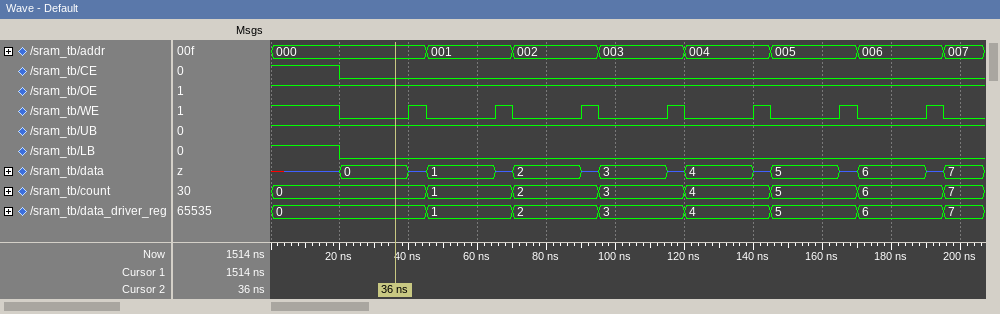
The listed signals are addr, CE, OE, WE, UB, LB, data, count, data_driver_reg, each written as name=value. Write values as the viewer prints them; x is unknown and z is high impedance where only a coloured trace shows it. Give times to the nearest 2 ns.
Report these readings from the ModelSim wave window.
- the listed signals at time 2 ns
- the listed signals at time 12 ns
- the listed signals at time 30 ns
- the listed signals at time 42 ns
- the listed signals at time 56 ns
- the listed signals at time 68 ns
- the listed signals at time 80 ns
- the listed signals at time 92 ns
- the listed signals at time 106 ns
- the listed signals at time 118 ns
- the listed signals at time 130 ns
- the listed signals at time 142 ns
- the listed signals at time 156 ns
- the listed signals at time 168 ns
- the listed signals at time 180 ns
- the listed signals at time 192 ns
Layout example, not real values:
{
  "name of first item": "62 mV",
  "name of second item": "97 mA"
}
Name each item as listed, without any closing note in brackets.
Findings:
{
  "the listed signals at time 2 ns": "addr=000, CE=1, OE=1, WE=1, UB=1, LB=1, data=x, count=0, data_driver_reg=0",
  "the listed signals at time 12 ns": "addr=000, CE=1, OE=1, WE=1, UB=1, LB=1, data=z, count=0, data_driver_reg=0",
  "the listed signals at time 30 ns": "addr=000, CE=0, OE=1, WE=0, UB=1, LB=0, data=0, count=0, data_driver_reg=0",
  "the listed signals at time 42 ns": "addr=000, CE=0, OE=1, WE=1, UB=1, LB=0, data=z, count=0, data_driver_reg=0",
  "the listed signals at time 56 ns": "addr=001, CE=0, OE=1, WE=0, UB=1, LB=0, data=1, count=1, data_driver_reg=1",
  "the listed signals at time 68 ns": "addr=001, CE=0, OE=1, WE=1, UB=1, LB=0, data=z, count=1, data_driver_reg=1",
  "the listed signals at time 80 ns": "addr=002, CE=0, OE=1, WE=0, UB=1, LB=0, data=2, count=2, data_driver_reg=2",
  "the listed signals at time 92 ns": "addr=002, CE=0, OE=1, WE=1, UB=1, LB=0, data=z, count=2, data_driver_reg=2",
  "the listed signals at time 106 ns": "addr=003, CE=0, OE=1, WE=0, UB=1, LB=0, data=3, count=3, data_driver_reg=3",
  "the listed signals at time 118 ns": "addr=003, CE=0, OE=1, WE=1, UB=1, LB=0, data=z, count=3, data_driver_reg=3",
  "the listed signals at time 130 ns": "addr=004, CE=0, OE=1, WE=0, UB=1, LB=0, data=4, count=4, data_driver_reg=4",
  "the listed signals at time 142 ns": "addr=004, CE=0, OE=1, WE=1, UB=1, LB=0, data=z, count=4, data_driver_reg=4",
  "the listed signals at time 156 ns": "addr=005, CE=0, OE=1, WE=0, UB=1, LB=0, data=5, count=5, data_driver_reg=5",
  "the listed signals at time 168 ns": "addr=005, CE=0, OE=1, WE=1, UB=1, LB=0, data=z, count=5, data_driver_reg=5",
  "the listed signals at time 180 ns": "addr=006, CE=0, OE=1, WE=0, UB=1, LB=0, data=6, count=6, data_driver_reg=6",
  "the listed signals at time 192 ns": "addr=006, CE=0, OE=1, WE=1, UB=1, LB=0, data=z, count=6, data_driver_reg=6"
}
